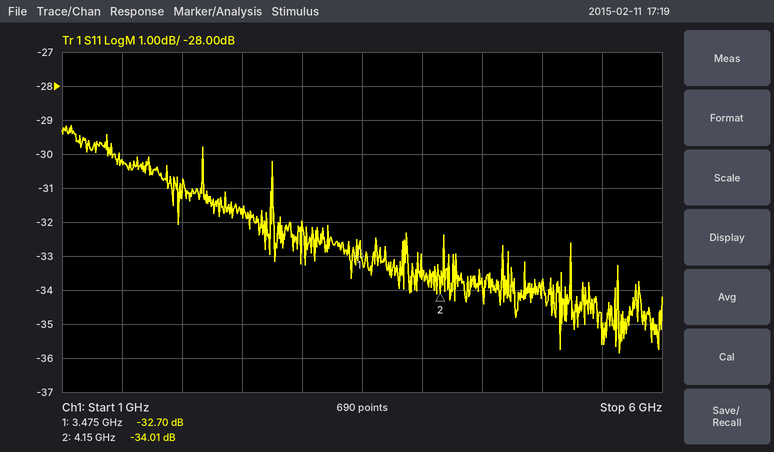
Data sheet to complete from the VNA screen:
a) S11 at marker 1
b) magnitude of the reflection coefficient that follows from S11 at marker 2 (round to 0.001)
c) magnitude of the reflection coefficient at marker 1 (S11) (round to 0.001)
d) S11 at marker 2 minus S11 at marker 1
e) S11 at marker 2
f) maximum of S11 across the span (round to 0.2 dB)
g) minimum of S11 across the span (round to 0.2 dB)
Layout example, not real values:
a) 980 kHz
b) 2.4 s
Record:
a) -32.70 dB
b) 0.020
c) 0.023
d) -1.31 dB
e) -34.01 dB
f) -29.2 dB
g) -35.8 dB
